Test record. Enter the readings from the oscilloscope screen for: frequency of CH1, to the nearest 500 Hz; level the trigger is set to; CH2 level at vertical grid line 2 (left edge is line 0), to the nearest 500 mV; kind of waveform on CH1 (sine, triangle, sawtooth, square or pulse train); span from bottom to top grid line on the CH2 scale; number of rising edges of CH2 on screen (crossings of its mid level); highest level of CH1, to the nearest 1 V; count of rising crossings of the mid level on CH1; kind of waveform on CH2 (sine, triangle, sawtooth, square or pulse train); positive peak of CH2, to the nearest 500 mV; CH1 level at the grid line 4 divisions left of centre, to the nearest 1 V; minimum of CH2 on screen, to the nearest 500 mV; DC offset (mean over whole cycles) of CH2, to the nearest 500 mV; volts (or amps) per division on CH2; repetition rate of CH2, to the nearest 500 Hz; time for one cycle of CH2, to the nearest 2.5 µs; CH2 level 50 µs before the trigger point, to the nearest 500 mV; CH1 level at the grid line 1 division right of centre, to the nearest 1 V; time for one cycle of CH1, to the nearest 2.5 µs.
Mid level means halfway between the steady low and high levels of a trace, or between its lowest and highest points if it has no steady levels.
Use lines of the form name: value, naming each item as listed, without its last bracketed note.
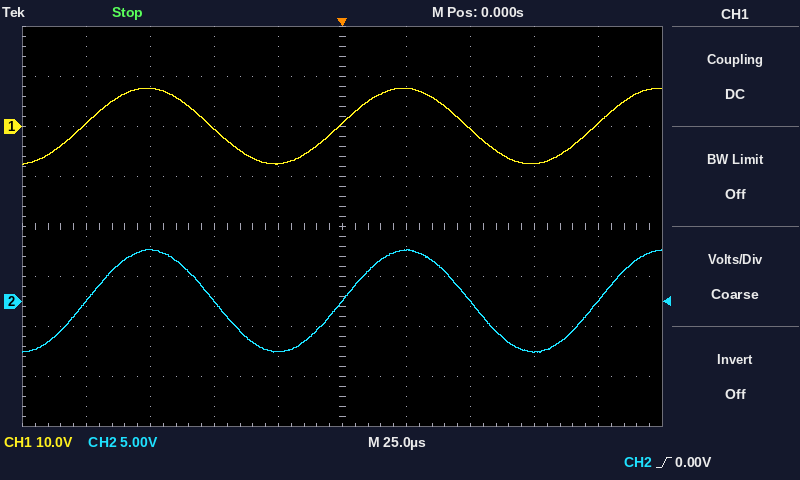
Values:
frequency of CH1, to the nearest 500 Hz: 10.0 kHz
level the trigger is set to: 0.00 V
CH2 level at vertical grid line 2 (left edge is line 0), to the nearest 500 mV: 5.0 V
kind of waveform on CH1: sine
span from bottom to top grid line on the CH2 scale: 40 V
number of rising edges of CH2 on screen: 3
highest level of CH1, to the nearest 1 V: 8 V
count of rising crossings of the mid level on CH1: 3
kind of waveform on CH2: sine
positive peak of CH2, to the nearest 500 mV: 5.0 V
CH1 level at the grid line 4 divisions left of centre, to the nearest 1 V: 1 V
minimum of CH2 on screen, to the nearest 500 mV: -5.0 V
DC offset (mean over whole cycles) of CH2, to the nearest 500 mV: 0.0 V
volts (or amps) per division on CH2: 5 V
repetition rate of CH2, to the nearest 500 Hz: 10.0 kHz
time for one cycle of CH2, to the nearest 2.5 µs: 100.0 µs
CH2 level 50 µs before the trigger point, to the nearest 500 mV: 0.0 V
CH1 level at the grid line 1 division right of centre, to the nearest 1 V: 8 V
time for one cycle of CH1, to the nearest 2.5 µs: 100.0 µs
